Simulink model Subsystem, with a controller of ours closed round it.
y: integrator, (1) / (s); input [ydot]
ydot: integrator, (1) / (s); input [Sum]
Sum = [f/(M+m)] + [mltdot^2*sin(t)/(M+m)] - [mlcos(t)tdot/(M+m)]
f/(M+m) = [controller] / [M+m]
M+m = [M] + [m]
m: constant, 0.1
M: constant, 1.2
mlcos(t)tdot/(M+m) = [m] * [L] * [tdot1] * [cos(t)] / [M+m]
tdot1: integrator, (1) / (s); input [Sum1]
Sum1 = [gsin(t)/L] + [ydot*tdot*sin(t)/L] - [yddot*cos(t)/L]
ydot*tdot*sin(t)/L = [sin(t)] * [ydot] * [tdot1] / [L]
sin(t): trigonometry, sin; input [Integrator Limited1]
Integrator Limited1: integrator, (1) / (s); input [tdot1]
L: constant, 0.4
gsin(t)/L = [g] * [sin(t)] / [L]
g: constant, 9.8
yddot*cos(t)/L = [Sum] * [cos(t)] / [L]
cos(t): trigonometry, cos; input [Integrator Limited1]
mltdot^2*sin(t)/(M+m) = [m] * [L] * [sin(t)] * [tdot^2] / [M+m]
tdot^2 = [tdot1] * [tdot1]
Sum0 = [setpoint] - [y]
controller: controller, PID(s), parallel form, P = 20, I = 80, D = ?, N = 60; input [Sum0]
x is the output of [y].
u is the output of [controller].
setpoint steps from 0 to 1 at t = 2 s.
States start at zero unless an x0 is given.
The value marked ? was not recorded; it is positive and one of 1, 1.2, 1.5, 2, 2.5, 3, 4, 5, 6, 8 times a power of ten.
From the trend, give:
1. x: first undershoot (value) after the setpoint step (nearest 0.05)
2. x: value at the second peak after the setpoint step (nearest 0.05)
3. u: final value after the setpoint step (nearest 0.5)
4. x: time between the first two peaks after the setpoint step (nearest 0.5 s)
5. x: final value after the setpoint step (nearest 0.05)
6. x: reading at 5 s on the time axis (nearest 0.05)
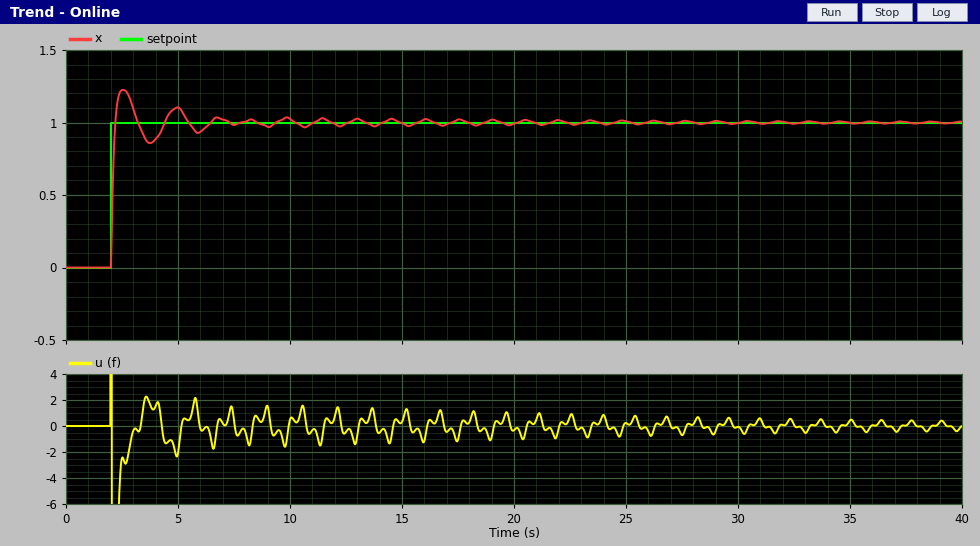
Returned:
0.85
1.10
0.0
2.5 s
1.00
1.10
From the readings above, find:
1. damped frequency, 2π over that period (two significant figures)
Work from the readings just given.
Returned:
2.5 rad/s
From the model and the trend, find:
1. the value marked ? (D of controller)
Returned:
12
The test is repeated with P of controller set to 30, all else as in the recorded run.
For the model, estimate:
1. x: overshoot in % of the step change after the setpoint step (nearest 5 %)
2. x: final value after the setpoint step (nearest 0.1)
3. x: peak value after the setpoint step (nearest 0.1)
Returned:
25 %
1.0
1.2
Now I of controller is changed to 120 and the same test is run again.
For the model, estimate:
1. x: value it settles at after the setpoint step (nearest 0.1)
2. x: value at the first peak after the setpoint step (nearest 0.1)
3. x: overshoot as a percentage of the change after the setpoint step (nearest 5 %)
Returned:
1.0
1.3
30 %
